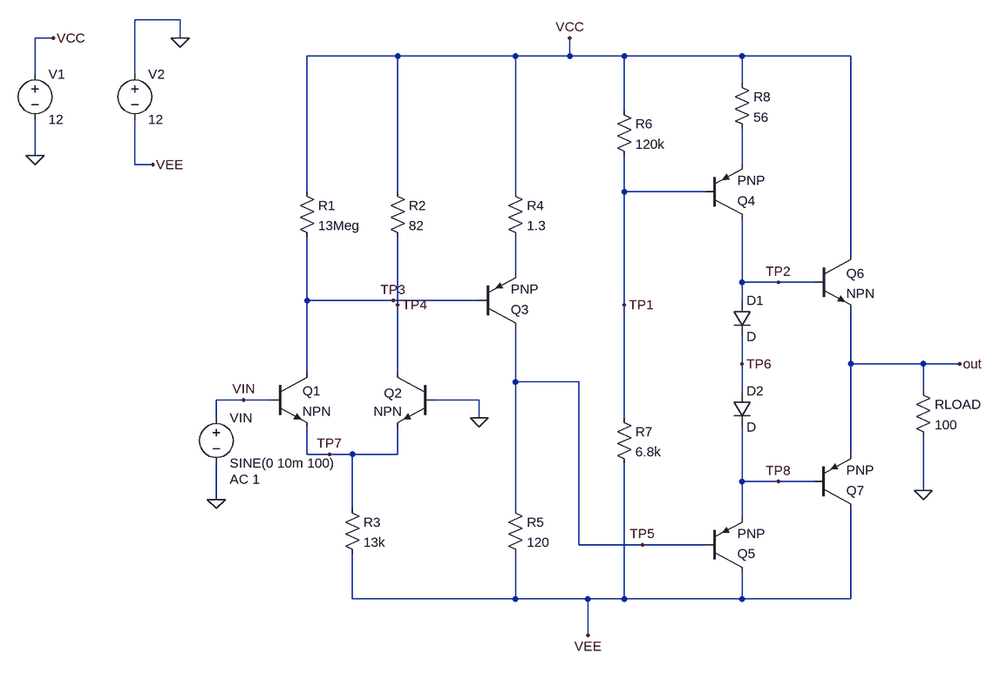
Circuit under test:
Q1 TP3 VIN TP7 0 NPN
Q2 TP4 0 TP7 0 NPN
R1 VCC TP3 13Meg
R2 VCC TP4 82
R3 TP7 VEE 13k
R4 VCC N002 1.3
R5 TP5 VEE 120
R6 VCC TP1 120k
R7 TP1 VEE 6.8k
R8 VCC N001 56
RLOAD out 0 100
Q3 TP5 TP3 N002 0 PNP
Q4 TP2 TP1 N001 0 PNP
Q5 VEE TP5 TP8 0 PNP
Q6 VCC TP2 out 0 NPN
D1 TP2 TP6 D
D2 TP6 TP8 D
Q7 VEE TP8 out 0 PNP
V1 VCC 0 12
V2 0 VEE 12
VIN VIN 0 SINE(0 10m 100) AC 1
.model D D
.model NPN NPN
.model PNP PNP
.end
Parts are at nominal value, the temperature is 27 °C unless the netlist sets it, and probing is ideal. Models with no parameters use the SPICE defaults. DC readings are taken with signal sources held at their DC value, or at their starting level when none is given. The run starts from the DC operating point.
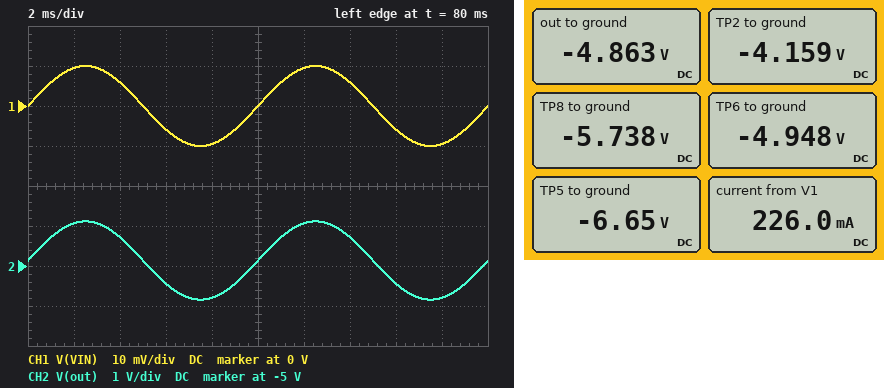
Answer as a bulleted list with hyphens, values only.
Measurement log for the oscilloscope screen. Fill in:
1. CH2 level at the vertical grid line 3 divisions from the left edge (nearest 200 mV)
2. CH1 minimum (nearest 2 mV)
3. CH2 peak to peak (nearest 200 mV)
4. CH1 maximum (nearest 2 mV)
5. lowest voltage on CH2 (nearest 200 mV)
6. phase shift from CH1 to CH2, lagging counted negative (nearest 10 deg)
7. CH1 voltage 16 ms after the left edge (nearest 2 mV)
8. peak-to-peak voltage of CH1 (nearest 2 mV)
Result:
- -5.4 V
- -10 mV
- 2.0 V
- 10 mV
- -5.8 V
- 0 deg
- -6 mV
- 20 mV
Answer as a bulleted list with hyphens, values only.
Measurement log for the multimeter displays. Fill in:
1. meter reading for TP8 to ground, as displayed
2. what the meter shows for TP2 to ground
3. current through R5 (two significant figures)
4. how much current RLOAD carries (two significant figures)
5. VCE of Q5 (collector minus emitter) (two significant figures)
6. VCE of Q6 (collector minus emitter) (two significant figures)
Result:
- -5.738 V
- -4.159 V
- 45 mA
- 49 mA
- -6.3 V
- 17 V
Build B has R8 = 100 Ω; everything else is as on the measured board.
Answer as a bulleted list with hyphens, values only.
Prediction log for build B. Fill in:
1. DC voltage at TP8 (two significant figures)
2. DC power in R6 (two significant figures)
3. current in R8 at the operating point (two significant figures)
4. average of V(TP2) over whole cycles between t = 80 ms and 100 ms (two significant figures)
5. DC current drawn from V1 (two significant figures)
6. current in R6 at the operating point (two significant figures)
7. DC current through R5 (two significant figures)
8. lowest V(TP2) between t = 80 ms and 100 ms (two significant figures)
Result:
- -5.8 V
- 1.7 mW
- 130 mA
- -4.2 V
- 180 mA
- 120 µA
- 44 mA
- -5.2 V
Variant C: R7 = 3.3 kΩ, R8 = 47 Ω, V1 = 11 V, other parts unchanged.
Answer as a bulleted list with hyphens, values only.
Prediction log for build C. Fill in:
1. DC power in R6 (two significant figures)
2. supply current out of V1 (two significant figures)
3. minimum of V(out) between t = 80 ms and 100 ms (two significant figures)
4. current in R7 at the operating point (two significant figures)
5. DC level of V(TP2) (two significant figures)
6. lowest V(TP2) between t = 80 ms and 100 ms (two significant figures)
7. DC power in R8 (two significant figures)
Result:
- 1.6 mW
- 320 mA
- -5.7 V
- 2.8 mA
- -4.0 V
- -5.0 V
- 3.5 W
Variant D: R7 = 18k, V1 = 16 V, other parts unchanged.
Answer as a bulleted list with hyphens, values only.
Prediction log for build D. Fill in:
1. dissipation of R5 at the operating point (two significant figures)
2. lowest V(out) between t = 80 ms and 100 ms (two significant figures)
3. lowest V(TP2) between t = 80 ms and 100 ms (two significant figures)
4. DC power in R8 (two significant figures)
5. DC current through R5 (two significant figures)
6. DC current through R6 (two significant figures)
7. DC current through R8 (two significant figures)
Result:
- 230 mW
- -5.9 V
- -5.3 V
- 690 mW
- 44 mA
- 59 µA
- 110 mA
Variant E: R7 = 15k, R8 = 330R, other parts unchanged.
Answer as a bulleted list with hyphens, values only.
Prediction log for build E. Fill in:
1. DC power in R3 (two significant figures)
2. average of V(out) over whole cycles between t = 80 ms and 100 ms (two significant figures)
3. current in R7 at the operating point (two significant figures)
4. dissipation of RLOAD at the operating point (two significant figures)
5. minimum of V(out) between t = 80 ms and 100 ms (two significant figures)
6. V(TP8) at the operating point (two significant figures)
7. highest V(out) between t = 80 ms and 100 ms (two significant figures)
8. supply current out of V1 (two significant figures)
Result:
- 9.7 mW
- -5.1 V
- 570 µA
- 260 mW
- -6.0 V
- -5.9 V
- -4.1 V
- 88 mA
